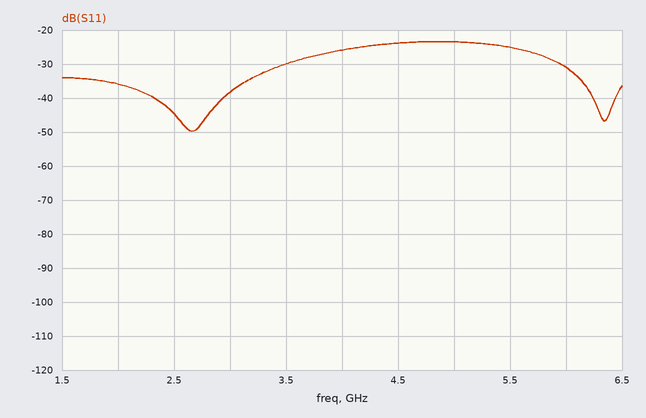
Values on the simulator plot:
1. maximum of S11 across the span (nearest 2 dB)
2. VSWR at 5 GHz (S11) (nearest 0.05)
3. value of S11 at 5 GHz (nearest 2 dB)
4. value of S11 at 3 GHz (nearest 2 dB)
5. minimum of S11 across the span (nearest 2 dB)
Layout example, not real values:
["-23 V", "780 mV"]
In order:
["-24 dB", "1.15", "-24 dB", "-38 dB", "-50 dB"]
